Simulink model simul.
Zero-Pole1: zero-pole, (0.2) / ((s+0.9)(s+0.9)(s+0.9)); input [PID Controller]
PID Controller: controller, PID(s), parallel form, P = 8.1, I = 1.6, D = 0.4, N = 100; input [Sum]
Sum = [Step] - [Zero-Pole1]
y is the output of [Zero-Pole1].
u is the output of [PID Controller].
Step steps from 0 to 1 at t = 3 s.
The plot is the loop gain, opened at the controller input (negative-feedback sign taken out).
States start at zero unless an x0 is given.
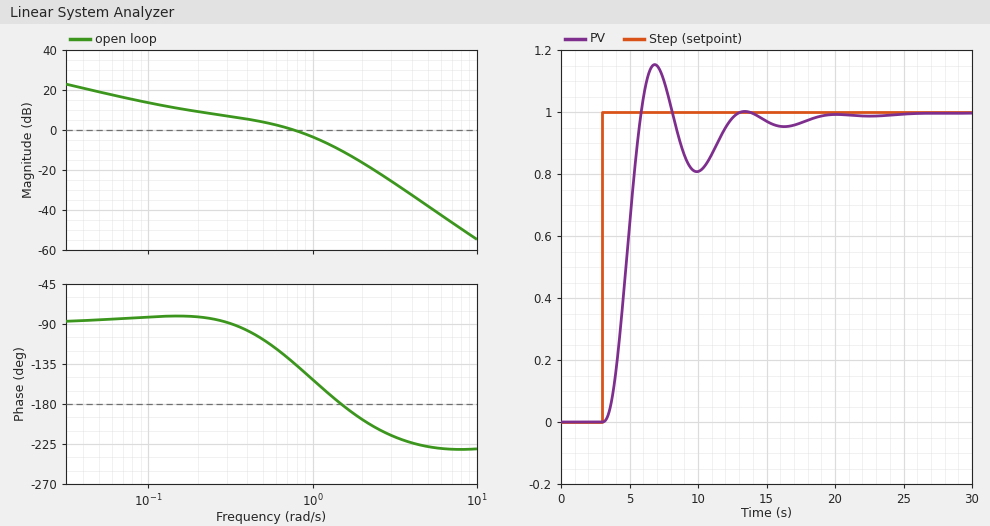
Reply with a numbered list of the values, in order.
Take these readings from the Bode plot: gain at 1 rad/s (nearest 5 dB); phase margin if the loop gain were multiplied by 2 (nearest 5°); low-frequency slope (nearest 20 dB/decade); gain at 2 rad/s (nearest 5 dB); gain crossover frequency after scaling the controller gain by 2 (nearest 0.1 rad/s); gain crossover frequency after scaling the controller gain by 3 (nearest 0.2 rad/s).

1. -5 dB
2. 15°
3. -20 dB/decade
4. -15 dB
5. 1.2 rad/s
6. 1.4 rad/s
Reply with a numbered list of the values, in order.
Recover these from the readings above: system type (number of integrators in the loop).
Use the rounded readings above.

1. 1
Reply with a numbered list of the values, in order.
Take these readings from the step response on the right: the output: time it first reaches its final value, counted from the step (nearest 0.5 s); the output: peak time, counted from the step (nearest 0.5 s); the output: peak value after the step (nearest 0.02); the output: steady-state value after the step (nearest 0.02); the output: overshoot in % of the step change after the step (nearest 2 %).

1. 3.0 s
2. 4.0 s
3. 1.16
4. 1.00
5. 16 %
